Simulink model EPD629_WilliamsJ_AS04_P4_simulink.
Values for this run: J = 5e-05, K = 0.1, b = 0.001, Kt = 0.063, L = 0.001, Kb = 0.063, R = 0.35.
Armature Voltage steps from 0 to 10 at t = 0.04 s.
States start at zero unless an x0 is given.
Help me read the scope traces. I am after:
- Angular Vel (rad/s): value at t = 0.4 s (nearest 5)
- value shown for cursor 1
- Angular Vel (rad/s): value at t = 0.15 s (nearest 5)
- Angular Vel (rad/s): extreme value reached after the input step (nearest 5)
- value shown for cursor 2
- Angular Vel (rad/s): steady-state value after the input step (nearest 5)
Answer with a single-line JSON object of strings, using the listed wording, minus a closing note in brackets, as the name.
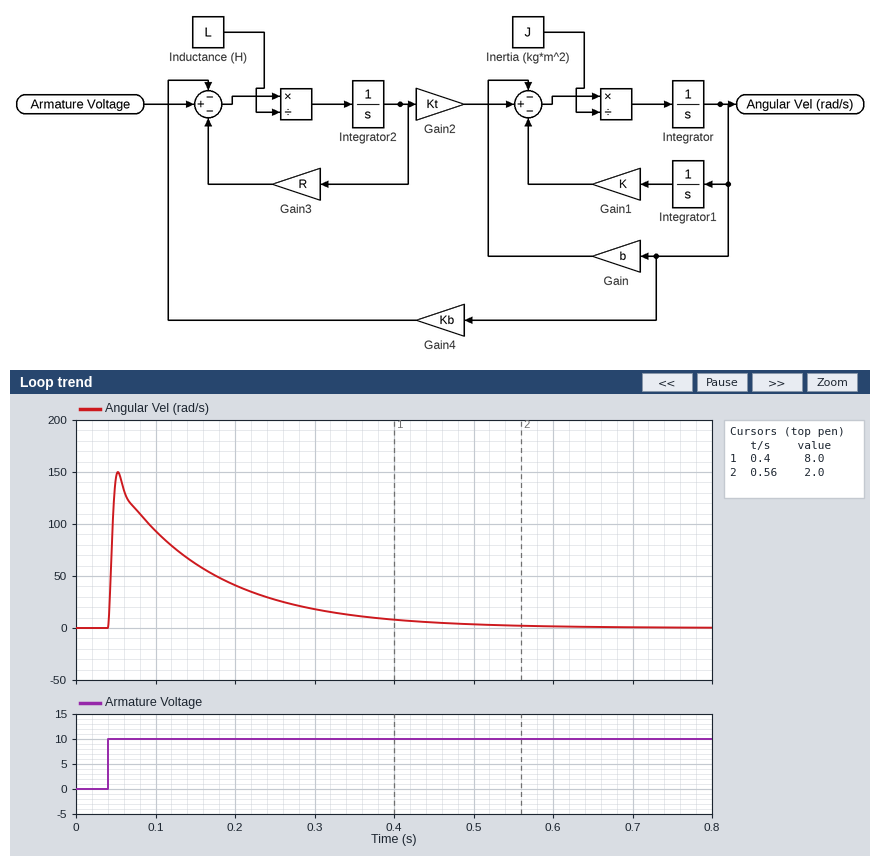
{"Angular Vel (rad/s): value at t = 0.4 s": "10", "value shown for cursor 1": "8.0", "Angular Vel (rad/s): value at t = 0.15 s": "60", "Angular Vel (rad/s): extreme value reached after the input step": "150", "value shown for cursor 2": "2.0", "Angular Vel (rad/s): steady-state value after the input step": "0"}
